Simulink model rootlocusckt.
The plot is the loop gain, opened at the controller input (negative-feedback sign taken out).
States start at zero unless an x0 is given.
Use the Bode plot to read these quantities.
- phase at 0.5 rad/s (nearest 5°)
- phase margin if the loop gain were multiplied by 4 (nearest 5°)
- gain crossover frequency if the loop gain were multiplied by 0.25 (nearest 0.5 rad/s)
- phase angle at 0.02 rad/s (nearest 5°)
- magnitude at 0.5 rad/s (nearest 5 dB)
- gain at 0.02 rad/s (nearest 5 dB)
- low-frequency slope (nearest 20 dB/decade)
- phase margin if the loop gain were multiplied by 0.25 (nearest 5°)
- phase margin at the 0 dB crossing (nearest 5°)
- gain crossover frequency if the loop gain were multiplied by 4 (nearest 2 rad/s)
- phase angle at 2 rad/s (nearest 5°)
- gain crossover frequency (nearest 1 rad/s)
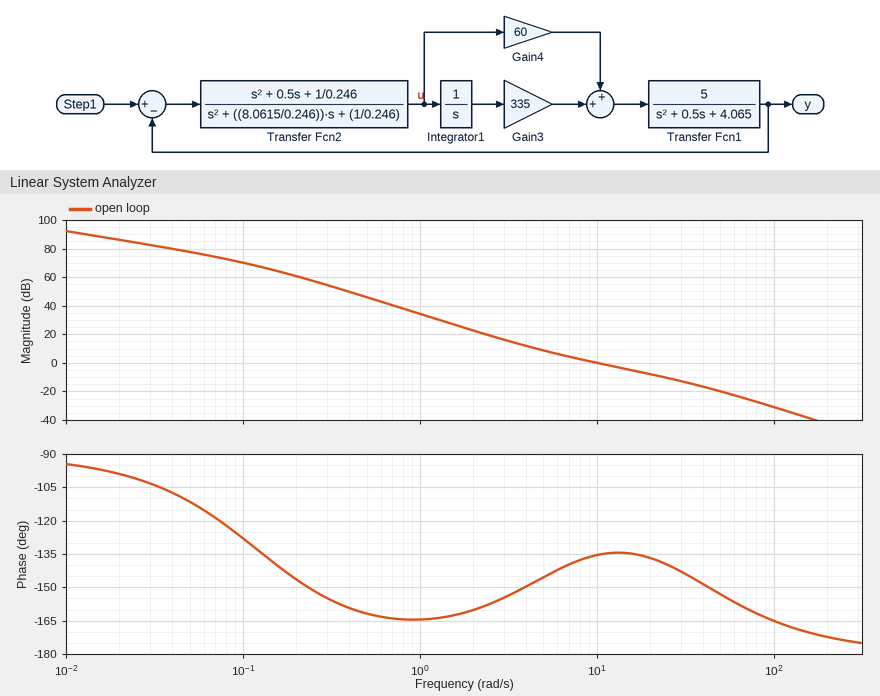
-160°
40°
4.0 rad/s
-100°
45 dB
85 dB
-20 dB/decade
30°
45°
28 rad/s
-160°
10 rad/s
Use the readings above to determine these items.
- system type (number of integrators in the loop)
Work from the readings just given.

1
